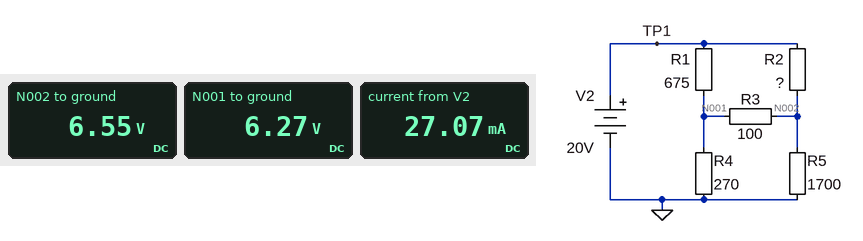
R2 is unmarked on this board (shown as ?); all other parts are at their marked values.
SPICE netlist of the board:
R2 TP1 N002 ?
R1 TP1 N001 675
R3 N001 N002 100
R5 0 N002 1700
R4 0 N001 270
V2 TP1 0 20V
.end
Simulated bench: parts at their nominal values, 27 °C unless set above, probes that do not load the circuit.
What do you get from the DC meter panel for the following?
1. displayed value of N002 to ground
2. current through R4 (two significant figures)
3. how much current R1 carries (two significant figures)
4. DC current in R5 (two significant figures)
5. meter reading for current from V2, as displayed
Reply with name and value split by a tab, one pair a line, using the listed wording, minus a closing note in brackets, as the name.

displayed value of N002 to ground	6.55 V
current through R4	23 mA
how much current R1 carries	20 mA
DC current in R5	3.9 mA
meter reading for current from V2, as displayed	27.07 mA
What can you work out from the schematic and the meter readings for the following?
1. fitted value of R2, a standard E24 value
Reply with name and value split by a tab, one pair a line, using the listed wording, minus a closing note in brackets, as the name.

fitted value of R2, a standard E24 value	2 kΩ
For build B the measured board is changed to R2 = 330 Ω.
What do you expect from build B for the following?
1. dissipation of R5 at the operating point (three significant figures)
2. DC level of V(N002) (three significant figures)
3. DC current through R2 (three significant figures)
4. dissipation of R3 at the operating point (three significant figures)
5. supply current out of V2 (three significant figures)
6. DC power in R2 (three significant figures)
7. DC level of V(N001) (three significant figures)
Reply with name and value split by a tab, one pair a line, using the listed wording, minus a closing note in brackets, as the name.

dissipation of R5 at the operating point	76.3 mW
DC level of V(N002)	11.4 V
DC current through R2	26.1 mA
dissipation of R3 at the operating point	37.6 mW
supply current out of V2	41.7 mA
DC power in R2	225 mW
DC level of V(N001)	9.45 V
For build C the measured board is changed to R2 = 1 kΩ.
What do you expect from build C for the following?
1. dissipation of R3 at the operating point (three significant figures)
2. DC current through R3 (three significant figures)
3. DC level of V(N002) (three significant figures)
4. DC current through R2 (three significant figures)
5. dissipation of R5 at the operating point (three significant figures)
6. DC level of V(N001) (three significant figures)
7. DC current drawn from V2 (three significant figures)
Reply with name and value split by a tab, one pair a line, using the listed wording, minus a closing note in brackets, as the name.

dissipation of R3 at the operating point	5.56 mW
DC current through R3	7.46 mA
DC level of V(N002)	7.90 V
DC current through R2	12.1 mA
dissipation of R5 at the operating point	36.7 mW
DC level of V(N001)	7.15 V
DC current drawn from V2	31.1 mA
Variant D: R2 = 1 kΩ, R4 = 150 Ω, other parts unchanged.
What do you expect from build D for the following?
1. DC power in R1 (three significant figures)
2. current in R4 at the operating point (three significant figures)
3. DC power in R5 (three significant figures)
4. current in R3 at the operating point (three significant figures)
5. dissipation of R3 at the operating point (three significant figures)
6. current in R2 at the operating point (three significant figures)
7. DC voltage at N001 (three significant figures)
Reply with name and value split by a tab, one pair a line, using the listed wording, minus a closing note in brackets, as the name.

DC power in R1	337 mW
current in R4 at the operating point	32.8 mA
DC power in R5	21.0 mW
current in R3 at the operating point	10.5 mA
dissipation of R3 at the operating point	11.0 mW
current in R2 at the operating point	14.0 mA
DC voltage at N001	4.93 V
